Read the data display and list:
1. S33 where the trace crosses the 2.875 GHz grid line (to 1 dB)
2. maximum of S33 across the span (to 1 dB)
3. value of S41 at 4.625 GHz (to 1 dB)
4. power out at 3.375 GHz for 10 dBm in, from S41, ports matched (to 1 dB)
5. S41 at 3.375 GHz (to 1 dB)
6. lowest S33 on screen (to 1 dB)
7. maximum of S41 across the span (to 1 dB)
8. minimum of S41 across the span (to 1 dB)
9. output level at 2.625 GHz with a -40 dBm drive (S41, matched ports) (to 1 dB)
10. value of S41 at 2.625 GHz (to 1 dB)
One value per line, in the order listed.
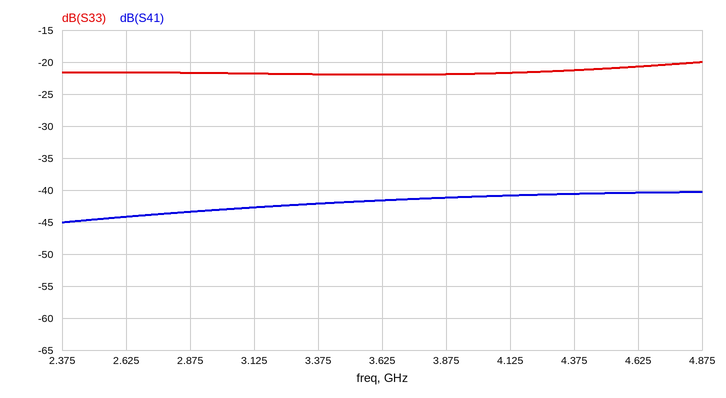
-22 dB
-20 dB
-40 dB
-32 dBm
-42 dB
-22 dB
-40 dB
-45 dB
-84 dBm
-44 dB
